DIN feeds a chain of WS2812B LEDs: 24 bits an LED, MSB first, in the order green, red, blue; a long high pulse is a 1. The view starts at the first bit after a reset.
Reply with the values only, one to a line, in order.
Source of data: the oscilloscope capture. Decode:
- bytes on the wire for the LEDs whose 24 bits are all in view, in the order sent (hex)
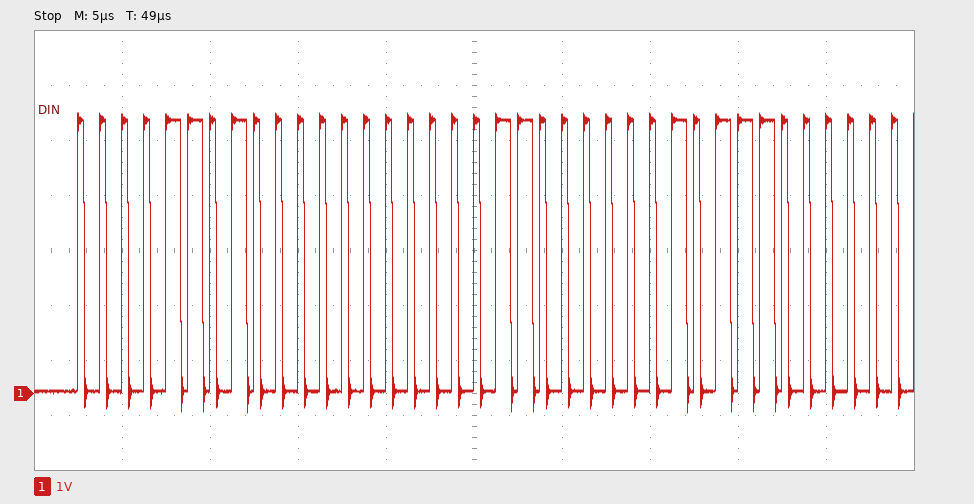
0D 00 18
